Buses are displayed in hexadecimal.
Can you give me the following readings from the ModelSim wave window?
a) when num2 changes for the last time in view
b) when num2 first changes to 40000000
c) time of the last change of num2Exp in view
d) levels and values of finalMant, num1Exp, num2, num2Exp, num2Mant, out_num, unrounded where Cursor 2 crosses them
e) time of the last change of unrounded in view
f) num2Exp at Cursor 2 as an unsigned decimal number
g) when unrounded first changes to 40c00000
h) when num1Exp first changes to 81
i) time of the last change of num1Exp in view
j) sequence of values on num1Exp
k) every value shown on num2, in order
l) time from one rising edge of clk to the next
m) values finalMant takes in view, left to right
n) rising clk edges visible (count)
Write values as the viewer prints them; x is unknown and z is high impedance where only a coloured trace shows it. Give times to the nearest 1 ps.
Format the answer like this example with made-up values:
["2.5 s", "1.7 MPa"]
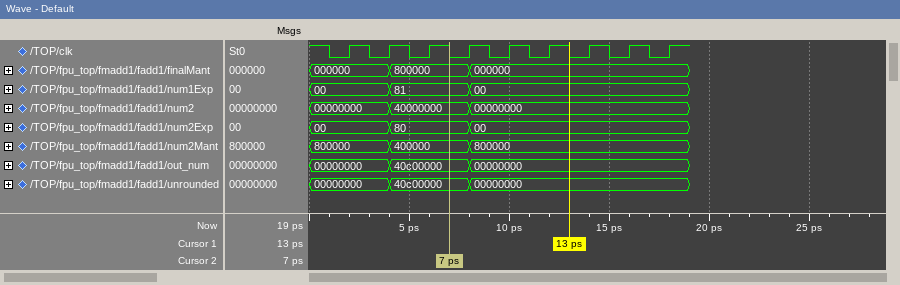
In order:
["8 ps", "4 ps", "8 ps", "finalMant=800000, num1Exp=81, num2=40000000, num2Exp=80, num2Mant=400000, out_num=40c00000, unrounded=40c00000", "8 ps", "128", "4 ps", "4 ps", "8 ps", "00, 81, 00", "00000000, 40000000, 00000000", "2 ps", "000000, 800000, 000000", "9"]
